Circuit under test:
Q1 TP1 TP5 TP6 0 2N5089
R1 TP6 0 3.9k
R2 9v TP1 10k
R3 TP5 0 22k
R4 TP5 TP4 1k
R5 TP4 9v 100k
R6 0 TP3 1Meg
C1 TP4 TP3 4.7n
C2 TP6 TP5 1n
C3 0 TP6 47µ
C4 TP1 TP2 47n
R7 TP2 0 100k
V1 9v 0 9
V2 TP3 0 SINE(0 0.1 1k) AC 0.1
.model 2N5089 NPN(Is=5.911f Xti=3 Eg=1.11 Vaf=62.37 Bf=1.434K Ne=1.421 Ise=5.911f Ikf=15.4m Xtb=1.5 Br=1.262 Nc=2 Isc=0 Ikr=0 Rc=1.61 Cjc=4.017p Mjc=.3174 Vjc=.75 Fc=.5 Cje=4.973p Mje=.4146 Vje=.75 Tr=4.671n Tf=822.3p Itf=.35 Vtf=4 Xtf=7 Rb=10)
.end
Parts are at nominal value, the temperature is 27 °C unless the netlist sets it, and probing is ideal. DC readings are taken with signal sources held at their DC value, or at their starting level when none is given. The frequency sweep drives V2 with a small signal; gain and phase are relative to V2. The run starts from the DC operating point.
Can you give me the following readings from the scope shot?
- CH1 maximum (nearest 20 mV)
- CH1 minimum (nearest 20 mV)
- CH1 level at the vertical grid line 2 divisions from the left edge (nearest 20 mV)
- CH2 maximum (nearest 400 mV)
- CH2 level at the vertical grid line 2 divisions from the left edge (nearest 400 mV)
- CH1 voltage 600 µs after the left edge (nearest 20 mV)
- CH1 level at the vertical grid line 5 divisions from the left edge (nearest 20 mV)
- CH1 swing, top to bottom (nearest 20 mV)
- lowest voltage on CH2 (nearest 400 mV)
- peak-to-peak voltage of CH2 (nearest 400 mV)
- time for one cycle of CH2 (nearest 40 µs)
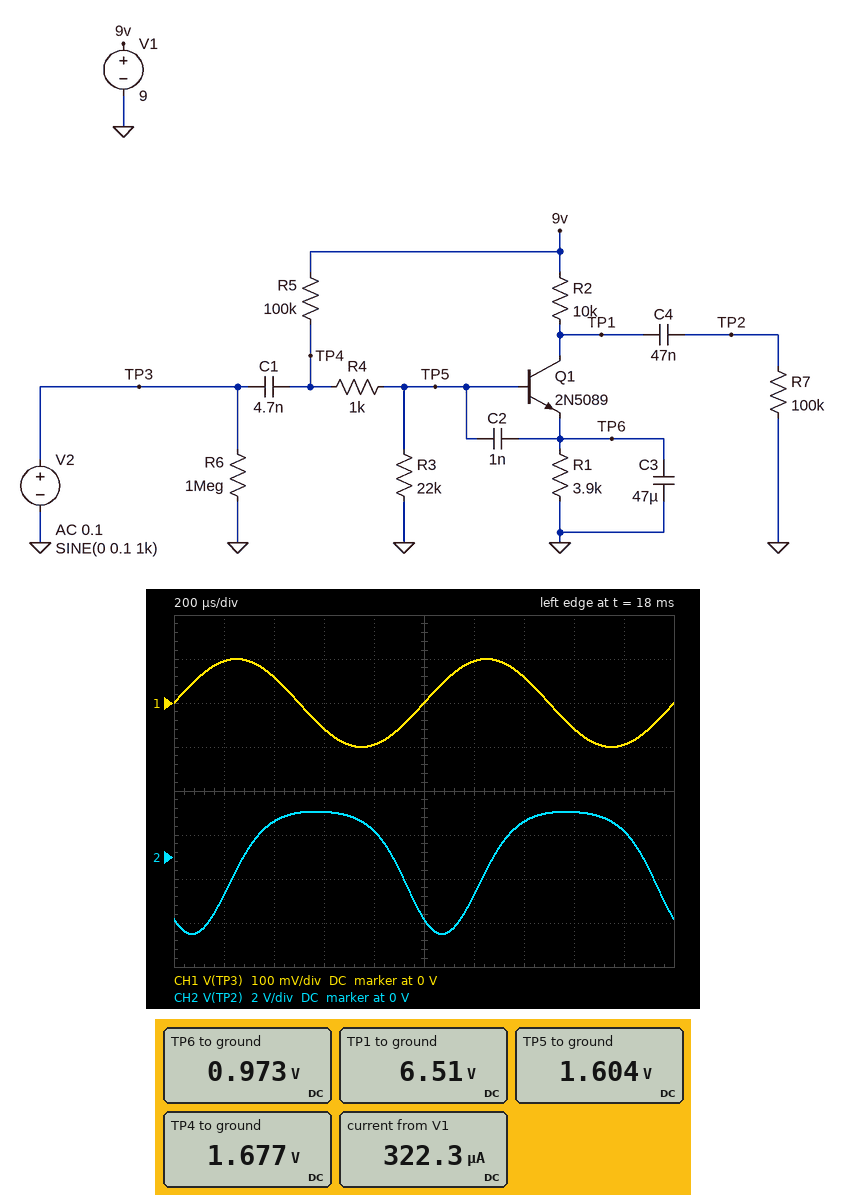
100 mV
-100 mV
60 mV
2.0 V
1.6 V
-60 mV
0 V
200 mV
-3.6 V
5.6 V
1.00 ms
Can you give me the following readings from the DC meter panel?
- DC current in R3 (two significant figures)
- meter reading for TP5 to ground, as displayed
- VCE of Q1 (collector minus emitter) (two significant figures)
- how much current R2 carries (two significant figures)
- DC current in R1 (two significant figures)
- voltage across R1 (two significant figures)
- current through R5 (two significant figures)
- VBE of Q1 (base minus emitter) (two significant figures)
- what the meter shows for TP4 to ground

73 µA
1.604 V
5.5 V
250 µA
250 µA
970 mV
73 µA
630 mV
1.677 V
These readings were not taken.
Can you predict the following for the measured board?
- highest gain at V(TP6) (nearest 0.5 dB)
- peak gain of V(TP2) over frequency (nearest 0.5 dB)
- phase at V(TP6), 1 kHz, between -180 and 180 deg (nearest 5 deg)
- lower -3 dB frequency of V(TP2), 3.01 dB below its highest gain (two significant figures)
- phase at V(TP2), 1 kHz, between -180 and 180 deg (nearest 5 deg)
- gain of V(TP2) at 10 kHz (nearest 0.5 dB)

-37.5 dB
36.0 dB
-30 deg
1.7 kHz
-115 deg
36.0 dB
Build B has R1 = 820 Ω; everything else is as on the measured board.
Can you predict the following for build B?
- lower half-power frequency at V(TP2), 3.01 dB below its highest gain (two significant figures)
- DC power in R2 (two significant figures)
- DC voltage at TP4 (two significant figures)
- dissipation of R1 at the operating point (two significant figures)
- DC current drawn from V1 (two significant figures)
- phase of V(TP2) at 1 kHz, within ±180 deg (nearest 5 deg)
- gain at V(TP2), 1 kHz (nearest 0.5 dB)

30 kHz
6.7 mW
1.4 V
570 µW
900 µA
-90 deg
-25.5 dB
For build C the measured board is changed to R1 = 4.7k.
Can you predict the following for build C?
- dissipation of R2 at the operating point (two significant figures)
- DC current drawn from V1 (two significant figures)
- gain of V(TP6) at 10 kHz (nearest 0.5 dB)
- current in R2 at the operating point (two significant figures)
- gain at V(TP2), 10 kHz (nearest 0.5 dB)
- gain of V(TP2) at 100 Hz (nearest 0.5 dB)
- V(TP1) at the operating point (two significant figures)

430 µW
280 µA
-54.0 dB
210 µA
34.5 dB
9.5 dB
6.9 V
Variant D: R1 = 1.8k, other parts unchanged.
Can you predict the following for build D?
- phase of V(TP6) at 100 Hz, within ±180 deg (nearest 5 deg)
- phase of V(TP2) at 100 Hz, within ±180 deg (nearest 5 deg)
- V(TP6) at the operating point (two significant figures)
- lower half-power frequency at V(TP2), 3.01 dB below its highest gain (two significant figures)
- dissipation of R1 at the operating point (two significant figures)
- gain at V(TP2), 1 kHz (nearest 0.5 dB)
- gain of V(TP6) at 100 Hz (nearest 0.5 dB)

20 deg
-50 deg
950 mV
1.9 kHz
500 µW
35.0 dB
-33.5 dB
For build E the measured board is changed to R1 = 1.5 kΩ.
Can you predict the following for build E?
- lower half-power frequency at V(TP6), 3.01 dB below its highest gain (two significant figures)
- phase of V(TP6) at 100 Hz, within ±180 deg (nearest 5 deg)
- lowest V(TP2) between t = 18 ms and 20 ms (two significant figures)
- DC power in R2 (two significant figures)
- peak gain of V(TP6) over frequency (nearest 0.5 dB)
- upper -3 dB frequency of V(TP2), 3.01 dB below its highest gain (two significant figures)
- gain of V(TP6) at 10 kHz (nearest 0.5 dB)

49 Hz
25 deg
-2.0 V
3.9 mW
-32.0 dB
140 kHz
-46.0 dB
